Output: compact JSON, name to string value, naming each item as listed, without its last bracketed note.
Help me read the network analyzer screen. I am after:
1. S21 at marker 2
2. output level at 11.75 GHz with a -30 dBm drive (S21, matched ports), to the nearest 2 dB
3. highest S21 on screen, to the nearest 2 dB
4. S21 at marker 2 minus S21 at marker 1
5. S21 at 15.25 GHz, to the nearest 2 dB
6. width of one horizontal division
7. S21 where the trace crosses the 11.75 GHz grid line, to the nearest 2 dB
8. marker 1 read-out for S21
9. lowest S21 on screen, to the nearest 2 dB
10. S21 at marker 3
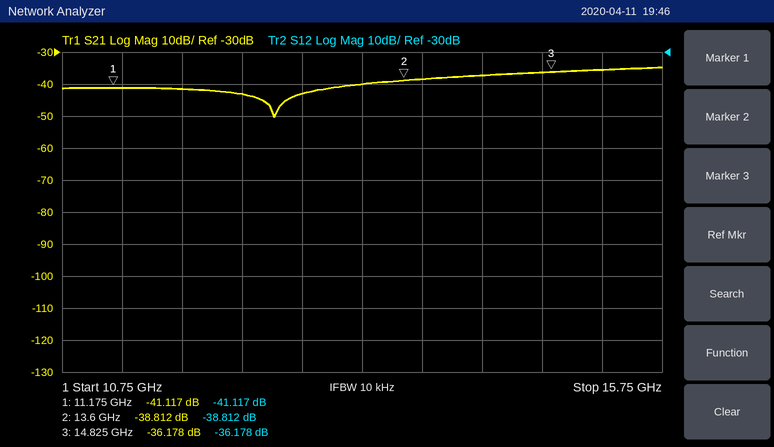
{"S21 at marker 2": "-38.812 dB", "output level at 11.75 GHz with a -30 dBm drive (S21, matched ports), to the nearest 2 dB": "-72 dBm", "highest S21 on screen, to the nearest 2 dB": "-34 dB", "S21 at marker 2 minus S21 at marker 1": "2.305 dB", "S21 at 15.25 GHz, to the nearest 2 dB": "-36 dB", "width of one horizontal division": "500 MHz", "S21 where the trace crosses the 11.75 GHz grid line, to the nearest 2 dB": "-42 dB", "marker 1 read-out for S21": "-41.117 dB", "lowest S21 on screen, to the nearest 2 dB": "-50 dB", "S21 at marker 3": "-36.178 dB"}
